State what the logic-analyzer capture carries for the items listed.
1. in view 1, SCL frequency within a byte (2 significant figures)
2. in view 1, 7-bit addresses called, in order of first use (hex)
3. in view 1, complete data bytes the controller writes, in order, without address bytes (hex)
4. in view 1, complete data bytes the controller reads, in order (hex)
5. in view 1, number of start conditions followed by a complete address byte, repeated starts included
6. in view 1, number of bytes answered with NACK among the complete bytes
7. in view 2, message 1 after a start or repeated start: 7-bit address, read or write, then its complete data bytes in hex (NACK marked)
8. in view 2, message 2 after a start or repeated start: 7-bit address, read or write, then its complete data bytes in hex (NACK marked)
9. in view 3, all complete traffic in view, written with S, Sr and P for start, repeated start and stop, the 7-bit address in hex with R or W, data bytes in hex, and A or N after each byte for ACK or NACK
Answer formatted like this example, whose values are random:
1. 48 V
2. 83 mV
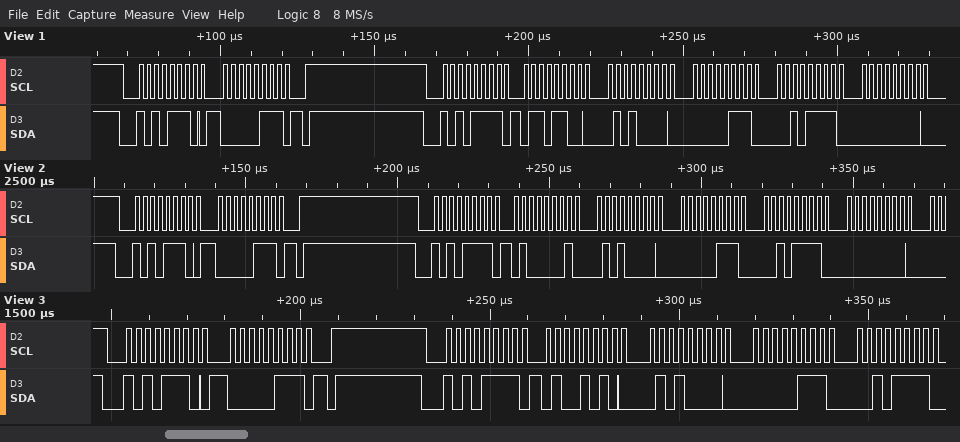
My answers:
1. 400 kHz
2. 0x57
3. 07
4. 6C 50 07 2F 00
5. 2
6. 0
7. 0x57 write: 07
8. 0x57 read: 41 50 07 2F 00
9. S 57W A 07 A P S 57R A 4A A 50 A 07 A 2F A
